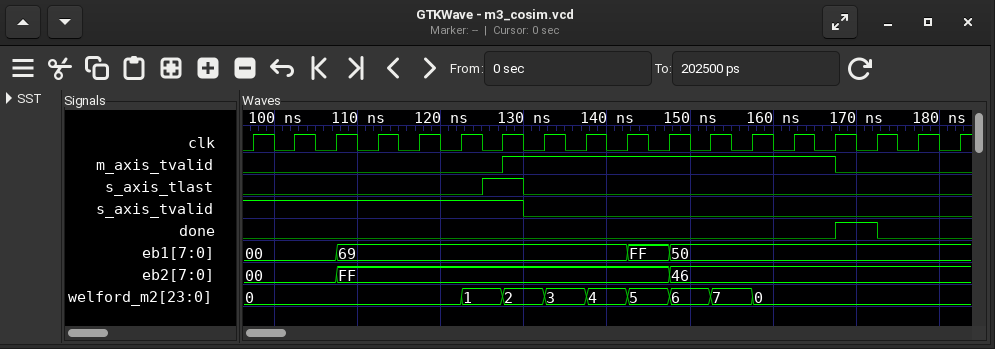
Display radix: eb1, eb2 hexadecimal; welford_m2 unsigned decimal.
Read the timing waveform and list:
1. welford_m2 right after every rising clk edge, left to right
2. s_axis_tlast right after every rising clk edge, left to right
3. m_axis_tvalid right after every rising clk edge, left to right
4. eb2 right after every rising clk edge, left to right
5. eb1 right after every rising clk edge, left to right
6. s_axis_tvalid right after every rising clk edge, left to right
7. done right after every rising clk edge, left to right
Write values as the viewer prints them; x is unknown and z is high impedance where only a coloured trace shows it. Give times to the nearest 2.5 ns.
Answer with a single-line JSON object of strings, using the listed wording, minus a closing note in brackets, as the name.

{"welford_m2 right after every rising clk edge, left to right": "0, 0, 0, 0, 0, 1, 2, 3, 4, 5, 6, 7, 0, 0, 0, 0, 0, 0", "s_axis_tlast right after every rising clk edge, left to right": "0 0 0 0 0 0 1 0 0 0 0 0 0 0 0 0 0 0", "m_axis_tvalid right after every rising clk edge, left to right": "0 0 0 0 0 0 1 1 1 1 1 1 1 1 0 0 0 0", "eb2 right after every rising clk edge, left to right": "00, 00, FF, FF, FF, FF, FF, FF, FF, FF, 46, 46, 46, 46, 46, 46, 46, 46", "eb1 right after every rising clk edge, left to right": "00, 00, 69, 69, 69, 69, 69, 69, 69, FF, 50, 50, 50, 50, 50, 50, 50, 50", "s_axis_tvalid right after every rising clk edge, left to right": "1 1 1 1 1 1 1 0 0 0 0 0 0 0 0 0 0 0", "done right after every rising clk edge, left to right": "0 0 0 0 0 0 0 0 0 0 0 0 0 0 1 0 0 0"}
